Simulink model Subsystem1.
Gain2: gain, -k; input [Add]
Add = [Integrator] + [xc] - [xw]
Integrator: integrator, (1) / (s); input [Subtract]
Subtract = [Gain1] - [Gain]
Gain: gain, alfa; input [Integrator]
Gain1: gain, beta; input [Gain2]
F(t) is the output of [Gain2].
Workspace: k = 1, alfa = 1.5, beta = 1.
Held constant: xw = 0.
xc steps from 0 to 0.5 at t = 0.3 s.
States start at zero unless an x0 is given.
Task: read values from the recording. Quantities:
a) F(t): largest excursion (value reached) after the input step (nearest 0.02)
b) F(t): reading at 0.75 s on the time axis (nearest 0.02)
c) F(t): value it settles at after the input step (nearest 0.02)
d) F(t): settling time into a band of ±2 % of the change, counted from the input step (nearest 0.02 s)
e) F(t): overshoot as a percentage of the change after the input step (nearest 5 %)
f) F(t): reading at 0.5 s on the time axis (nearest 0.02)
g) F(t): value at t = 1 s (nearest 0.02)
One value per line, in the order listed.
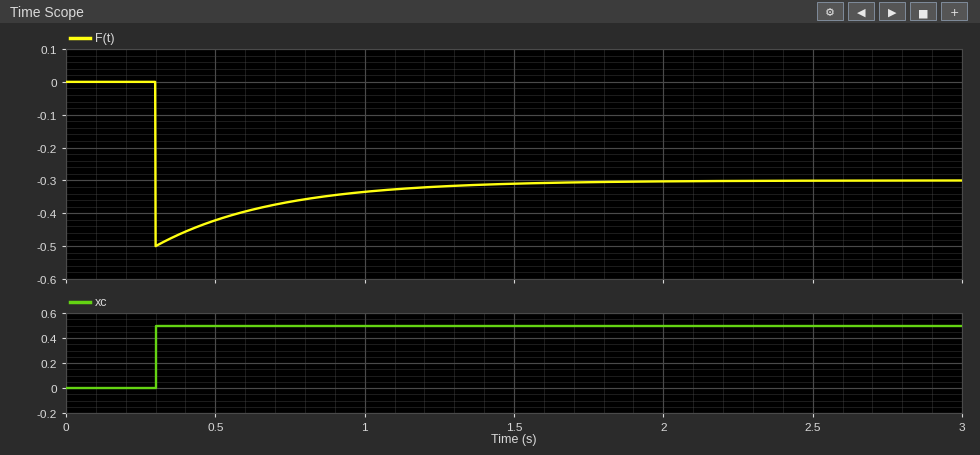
-0.50
-0.36
-0.30
1.40 s
65 %
-0.42
-0.34
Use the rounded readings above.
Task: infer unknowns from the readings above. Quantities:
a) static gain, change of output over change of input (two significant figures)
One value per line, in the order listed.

-0.60
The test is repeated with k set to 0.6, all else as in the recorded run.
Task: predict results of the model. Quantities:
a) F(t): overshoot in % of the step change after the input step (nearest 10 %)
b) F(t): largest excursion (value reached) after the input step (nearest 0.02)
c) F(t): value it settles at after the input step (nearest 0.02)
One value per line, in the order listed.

40 %
-0.30
-0.22
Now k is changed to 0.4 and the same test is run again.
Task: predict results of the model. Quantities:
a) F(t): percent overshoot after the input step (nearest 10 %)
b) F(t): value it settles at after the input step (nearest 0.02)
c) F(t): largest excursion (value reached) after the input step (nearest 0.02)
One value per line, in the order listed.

30 %
-0.16
-0.20
